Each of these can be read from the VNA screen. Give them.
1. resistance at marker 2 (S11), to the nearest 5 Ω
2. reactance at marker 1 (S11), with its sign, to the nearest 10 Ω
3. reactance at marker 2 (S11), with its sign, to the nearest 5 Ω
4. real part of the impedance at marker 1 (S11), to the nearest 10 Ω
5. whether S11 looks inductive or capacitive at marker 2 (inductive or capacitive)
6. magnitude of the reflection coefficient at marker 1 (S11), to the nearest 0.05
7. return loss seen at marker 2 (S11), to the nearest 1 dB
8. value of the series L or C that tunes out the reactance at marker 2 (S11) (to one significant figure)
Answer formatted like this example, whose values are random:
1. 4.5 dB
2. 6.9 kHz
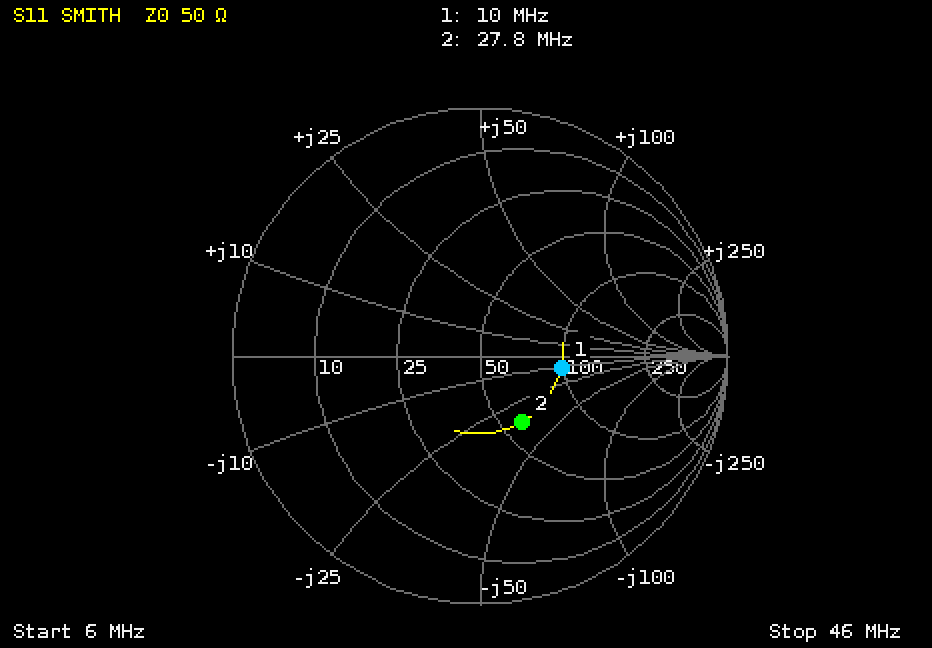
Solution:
1. 60 Ω
2. -10 Ω
3. -35 Ω
4. 100 Ω
5. capacitive
6. 0.35
7. 10 dB
8. 200 nH
